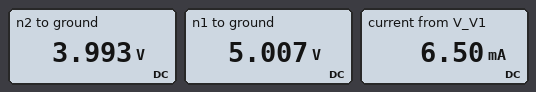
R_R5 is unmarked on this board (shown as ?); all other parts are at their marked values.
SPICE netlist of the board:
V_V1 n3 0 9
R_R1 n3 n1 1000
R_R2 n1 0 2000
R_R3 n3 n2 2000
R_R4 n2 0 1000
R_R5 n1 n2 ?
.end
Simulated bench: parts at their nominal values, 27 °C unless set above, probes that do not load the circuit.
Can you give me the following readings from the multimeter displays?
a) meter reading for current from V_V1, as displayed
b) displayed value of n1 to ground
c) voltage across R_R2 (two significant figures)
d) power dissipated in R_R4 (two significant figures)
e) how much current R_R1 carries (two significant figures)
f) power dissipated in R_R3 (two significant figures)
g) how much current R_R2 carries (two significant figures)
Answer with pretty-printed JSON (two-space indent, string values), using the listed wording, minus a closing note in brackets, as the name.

{
  "meter reading for current from V_V1, as displayed": "6.50 mA",
  "displayed value of n1 to ground": "5.007 V",
  "voltage across R_R2": "5.0 V",
  "power dissipated in R_R4": "16 mW",
  "how much current R_R1 carries": "4.0 mA",
  "power dissipated in R_R3": "13 mW",
  "how much current R_R2 carries": "2.5 mA"
}
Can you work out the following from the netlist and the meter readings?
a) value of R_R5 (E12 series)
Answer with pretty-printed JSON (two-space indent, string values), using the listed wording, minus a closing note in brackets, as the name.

{
  "value of R_R5": "680 Ω"
}
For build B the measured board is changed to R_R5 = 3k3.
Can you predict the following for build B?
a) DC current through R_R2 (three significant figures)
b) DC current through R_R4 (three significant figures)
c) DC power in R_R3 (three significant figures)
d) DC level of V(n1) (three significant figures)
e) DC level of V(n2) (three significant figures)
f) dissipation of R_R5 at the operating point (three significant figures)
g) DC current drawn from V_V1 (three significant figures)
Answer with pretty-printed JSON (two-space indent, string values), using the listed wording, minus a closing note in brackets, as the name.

{
  "DC current through R_R2": "2.78 mA",
  "DC current through R_R4": "3.43 mA",
  "DC power in R_R3": "15.5 mW",
  "DC level of V(n1)": "5.57 V",
  "DC level of V(n2)": "3.43 V",
  "dissipation of R_R5 at the operating point": "1.38 mW",
  "DC current drawn from V_V1": "6.22 mA"
}
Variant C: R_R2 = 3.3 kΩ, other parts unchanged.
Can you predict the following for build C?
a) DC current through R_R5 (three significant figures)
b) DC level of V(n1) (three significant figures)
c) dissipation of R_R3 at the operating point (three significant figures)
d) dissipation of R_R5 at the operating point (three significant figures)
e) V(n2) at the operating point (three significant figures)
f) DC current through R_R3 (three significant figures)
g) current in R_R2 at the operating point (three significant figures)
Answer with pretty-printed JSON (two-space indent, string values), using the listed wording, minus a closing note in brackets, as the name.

{
  "DC current through R_R5": "1.85 mA",
  "DC level of V(n1)": "5.49 V",
  "dissipation of R_R3 at the operating point": "11.4 mW",
  "dissipation of R_R5 at the operating point": "2.32 mW",
  "V(n2) at the operating point": "4.23 V",
  "DC current through R_R3": "2.38 mA",
  "current in R_R2 at the operating point": "1.66 mA"
}
